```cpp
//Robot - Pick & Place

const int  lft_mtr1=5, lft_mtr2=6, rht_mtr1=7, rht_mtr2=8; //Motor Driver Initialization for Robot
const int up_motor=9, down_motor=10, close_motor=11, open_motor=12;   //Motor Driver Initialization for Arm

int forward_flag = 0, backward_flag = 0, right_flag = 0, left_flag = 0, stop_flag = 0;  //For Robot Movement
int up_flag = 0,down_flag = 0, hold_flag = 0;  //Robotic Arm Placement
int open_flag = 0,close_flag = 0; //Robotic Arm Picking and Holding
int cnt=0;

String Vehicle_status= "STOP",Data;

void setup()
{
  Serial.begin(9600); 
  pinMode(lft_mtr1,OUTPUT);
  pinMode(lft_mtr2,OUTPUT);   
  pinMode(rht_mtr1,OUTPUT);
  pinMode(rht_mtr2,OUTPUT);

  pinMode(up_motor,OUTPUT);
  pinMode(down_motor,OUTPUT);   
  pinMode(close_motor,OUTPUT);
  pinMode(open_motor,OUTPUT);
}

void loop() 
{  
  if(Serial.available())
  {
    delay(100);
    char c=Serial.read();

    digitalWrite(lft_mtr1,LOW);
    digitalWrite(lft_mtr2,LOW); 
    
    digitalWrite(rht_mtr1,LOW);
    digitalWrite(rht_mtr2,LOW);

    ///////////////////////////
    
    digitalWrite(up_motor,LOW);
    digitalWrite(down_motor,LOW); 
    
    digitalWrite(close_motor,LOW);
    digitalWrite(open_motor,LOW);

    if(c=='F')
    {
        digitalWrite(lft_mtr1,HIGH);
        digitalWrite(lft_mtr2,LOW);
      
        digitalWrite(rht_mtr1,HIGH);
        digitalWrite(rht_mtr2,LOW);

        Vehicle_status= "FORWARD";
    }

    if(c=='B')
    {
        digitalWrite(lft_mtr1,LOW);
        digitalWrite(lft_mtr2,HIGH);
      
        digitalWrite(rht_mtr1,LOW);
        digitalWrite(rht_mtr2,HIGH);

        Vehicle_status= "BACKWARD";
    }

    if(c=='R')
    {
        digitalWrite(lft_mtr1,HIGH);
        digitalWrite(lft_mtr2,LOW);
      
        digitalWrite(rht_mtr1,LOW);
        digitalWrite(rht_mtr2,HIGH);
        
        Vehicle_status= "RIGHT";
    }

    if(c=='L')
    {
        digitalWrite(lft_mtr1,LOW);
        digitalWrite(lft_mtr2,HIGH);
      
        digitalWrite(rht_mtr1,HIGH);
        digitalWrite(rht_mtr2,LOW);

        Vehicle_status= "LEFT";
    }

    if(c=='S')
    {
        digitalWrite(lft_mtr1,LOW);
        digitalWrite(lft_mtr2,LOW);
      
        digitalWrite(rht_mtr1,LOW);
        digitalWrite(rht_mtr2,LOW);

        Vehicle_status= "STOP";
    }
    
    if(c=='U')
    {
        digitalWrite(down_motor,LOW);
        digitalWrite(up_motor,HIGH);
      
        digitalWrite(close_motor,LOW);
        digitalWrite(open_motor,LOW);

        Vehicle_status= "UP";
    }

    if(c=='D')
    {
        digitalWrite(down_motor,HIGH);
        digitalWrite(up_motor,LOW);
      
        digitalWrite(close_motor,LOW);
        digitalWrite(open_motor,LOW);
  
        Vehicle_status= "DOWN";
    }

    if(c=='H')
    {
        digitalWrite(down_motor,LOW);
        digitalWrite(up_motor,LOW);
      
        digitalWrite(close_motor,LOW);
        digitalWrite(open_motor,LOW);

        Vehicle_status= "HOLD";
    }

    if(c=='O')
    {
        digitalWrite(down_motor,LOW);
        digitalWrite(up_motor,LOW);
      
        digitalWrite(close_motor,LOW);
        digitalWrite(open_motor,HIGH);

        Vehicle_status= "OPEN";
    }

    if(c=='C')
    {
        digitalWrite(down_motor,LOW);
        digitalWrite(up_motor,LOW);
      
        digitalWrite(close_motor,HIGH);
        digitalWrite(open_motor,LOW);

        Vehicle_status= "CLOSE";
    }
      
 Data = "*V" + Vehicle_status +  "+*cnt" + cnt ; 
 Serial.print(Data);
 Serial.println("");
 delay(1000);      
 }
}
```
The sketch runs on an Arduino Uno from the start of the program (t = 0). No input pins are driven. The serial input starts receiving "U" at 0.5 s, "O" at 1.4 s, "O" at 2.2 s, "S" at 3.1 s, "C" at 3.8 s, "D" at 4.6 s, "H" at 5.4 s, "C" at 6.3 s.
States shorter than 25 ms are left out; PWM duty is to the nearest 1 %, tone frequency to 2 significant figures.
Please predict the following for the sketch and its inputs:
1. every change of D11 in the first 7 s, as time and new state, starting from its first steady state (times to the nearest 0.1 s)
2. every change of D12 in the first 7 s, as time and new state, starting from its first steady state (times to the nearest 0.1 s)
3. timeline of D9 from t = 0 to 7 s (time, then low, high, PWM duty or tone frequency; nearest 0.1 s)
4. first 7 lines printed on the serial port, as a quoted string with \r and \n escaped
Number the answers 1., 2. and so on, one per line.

1. 0 s low; 5 s high; 6.1 s low
2. 0 s low; 1.7 s high; 3.9 s low
3. 0 s low; 0.6 s high; 1.7 s low
4. "*VUP+*cnt0\r\n*VOPEN+*cnt0\r\n*VOPEN+*cnt0\r\n*VSTOP+*cnt0\r\n*VCLOSE+*cnt0\r\n*VDOWN+*cnt0\r\n*VHOLD+*cnt0\r\n"
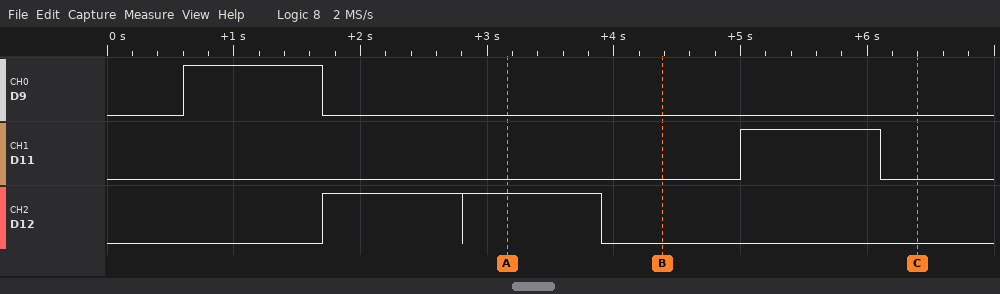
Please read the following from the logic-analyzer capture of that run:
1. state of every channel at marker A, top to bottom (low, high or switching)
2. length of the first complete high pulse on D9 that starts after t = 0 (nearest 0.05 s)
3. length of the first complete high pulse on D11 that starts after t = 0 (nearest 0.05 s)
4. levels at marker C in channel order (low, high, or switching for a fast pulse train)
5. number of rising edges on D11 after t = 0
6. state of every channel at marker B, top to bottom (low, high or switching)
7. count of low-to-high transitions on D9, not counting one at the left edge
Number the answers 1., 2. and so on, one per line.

1. D9 low, D11 low, D12 high
2. 1.10 s
3. 1.10 s
4. D9 low, D11 low, D12 low
5. 1
6. D9 low, D11 low, D12 low
7. 1
